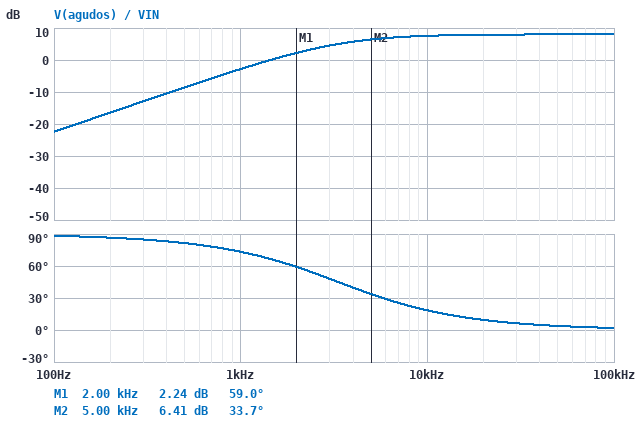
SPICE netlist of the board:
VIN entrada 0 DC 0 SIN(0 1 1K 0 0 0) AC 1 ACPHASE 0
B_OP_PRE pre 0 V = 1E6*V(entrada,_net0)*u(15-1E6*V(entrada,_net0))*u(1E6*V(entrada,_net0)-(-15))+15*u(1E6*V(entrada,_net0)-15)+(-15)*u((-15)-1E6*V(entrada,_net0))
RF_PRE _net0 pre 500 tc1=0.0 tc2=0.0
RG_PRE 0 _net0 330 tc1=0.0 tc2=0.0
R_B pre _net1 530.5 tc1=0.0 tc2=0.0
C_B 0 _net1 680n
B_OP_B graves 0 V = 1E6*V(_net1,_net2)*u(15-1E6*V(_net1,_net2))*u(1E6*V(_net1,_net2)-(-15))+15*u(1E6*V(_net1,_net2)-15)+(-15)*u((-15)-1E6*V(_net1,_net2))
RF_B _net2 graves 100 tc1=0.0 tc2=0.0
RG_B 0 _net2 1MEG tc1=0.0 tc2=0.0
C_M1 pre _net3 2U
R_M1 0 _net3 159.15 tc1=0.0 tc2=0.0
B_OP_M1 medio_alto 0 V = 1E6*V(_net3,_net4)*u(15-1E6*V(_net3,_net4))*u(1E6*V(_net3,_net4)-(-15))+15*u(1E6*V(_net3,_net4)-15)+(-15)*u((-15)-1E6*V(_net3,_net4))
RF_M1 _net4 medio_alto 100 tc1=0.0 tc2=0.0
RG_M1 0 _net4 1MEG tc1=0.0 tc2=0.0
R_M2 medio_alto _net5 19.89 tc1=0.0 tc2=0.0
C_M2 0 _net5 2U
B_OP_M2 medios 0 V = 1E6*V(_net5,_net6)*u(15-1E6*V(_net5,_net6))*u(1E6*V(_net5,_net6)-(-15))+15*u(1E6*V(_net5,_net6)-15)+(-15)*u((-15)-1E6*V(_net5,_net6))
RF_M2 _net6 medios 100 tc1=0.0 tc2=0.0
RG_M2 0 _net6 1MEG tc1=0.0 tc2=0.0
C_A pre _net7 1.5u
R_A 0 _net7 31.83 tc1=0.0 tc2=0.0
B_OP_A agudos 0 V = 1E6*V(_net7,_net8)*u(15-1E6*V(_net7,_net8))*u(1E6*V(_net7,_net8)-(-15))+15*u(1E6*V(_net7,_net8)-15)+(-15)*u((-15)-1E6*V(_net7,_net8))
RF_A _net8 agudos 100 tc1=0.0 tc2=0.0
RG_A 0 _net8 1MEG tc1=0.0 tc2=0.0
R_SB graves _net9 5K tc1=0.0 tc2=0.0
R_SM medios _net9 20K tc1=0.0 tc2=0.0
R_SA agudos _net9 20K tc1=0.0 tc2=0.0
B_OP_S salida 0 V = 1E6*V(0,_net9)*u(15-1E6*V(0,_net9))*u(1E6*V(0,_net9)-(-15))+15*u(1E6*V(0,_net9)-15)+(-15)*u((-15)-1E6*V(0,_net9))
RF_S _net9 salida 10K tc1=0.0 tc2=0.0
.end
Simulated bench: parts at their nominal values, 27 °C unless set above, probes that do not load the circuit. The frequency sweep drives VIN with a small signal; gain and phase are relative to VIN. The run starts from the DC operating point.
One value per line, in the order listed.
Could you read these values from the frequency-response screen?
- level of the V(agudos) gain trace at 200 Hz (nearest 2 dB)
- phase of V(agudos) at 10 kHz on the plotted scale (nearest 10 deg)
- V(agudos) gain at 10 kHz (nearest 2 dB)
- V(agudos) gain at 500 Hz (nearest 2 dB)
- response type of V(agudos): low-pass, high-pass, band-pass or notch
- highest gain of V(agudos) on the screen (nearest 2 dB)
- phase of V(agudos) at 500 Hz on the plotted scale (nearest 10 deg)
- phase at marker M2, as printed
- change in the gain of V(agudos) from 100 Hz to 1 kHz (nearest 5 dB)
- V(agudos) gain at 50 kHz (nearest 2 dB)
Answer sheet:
-16 dB
20 deg
8 dB
-8 dB
high-pass
8 dB
80 deg
33.7 deg
20 dB
8 dB
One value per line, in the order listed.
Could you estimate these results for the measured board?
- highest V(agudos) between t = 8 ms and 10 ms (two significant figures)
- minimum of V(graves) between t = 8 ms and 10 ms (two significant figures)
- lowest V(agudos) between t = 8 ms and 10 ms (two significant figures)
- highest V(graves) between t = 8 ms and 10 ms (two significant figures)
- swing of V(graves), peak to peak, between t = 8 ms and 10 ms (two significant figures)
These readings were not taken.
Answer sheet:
720 mV
-1.0 V
-720 mV
1.0 V
2.0 V
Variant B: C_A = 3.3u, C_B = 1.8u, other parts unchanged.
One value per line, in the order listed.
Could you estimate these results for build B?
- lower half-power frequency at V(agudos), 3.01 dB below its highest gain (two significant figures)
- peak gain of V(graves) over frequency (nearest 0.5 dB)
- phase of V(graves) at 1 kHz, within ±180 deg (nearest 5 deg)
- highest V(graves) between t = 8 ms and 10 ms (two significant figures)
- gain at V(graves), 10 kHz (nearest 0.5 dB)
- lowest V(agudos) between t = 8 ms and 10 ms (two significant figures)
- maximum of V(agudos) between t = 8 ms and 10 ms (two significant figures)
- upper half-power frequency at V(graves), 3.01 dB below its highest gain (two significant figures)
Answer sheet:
1.5 kHz
8.0 dB
-80 deg
410 mV
-27.5 dB
-1.4 V
1.4 V
170 Hz
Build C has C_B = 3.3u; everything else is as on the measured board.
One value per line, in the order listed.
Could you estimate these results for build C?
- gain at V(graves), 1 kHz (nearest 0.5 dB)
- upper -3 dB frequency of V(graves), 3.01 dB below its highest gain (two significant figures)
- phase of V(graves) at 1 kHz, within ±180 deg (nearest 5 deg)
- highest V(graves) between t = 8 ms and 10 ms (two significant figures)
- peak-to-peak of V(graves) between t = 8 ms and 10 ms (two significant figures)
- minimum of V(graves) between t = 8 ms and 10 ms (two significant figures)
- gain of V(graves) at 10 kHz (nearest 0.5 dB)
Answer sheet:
-13.0 dB
91 Hz
-85 deg
230 mV
460 mV
-230 mV
-33.0 dB
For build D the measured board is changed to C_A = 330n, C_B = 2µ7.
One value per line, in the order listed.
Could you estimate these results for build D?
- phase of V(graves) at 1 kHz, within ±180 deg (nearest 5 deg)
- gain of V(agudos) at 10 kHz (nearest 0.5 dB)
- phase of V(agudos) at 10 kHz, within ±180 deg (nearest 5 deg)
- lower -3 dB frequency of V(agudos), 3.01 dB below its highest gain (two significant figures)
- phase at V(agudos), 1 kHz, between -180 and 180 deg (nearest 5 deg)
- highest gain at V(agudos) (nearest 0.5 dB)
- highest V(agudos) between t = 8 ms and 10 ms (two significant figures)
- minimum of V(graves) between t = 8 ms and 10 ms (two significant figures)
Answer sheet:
-85 deg
3.0 dB
55 deg
15 kHz
85 deg
8.0 dB
170 mV
-280 mV
